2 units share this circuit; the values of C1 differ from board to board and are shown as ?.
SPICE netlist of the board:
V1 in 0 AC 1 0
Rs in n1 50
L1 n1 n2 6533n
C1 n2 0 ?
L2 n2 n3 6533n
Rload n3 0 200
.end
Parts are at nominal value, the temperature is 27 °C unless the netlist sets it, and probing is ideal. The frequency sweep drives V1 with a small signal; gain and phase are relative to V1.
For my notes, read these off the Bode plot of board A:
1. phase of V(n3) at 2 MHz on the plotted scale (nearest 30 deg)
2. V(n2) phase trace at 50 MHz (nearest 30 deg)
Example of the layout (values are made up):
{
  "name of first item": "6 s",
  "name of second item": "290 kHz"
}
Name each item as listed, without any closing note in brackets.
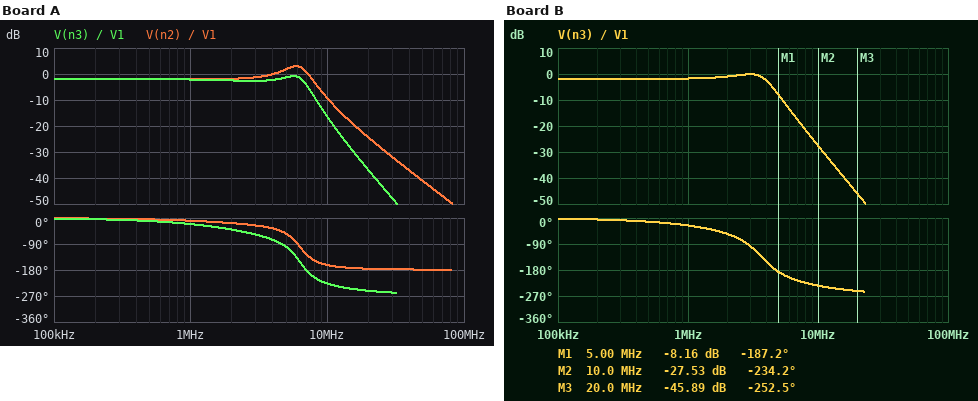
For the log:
{
  "phase of V(n3) at 2 MHz on the plotted scale": "-30 deg",
  "V(n2) phase trace at 50 MHz": "-180 deg"
}
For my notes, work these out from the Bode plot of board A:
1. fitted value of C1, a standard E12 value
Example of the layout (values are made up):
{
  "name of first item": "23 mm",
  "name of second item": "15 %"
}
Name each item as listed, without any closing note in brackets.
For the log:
{
  "fitted value of C1, a standard E12 value": "180 pF"
}
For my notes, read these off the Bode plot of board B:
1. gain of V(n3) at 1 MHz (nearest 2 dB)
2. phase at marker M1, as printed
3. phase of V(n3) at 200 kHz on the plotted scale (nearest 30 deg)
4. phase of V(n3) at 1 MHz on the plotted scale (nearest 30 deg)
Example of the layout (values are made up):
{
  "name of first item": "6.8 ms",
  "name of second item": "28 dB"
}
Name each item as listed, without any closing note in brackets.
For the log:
{
  "gain of V(n3) at 1 MHz": "-2 dB",
  "phase at marker M1, as printed": "-187.2 deg",
  "phase of V(n3) at 200 kHz on the plotted scale": "0 deg",
  "phase of V(n3) at 1 MHz on the plotted scale": "-30 deg"
}
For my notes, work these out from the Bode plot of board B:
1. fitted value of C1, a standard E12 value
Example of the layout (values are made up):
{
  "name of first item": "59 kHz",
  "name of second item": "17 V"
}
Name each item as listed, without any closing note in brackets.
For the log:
{
  "fitted value of C1, a standard E12 value": "470 pF"
}
